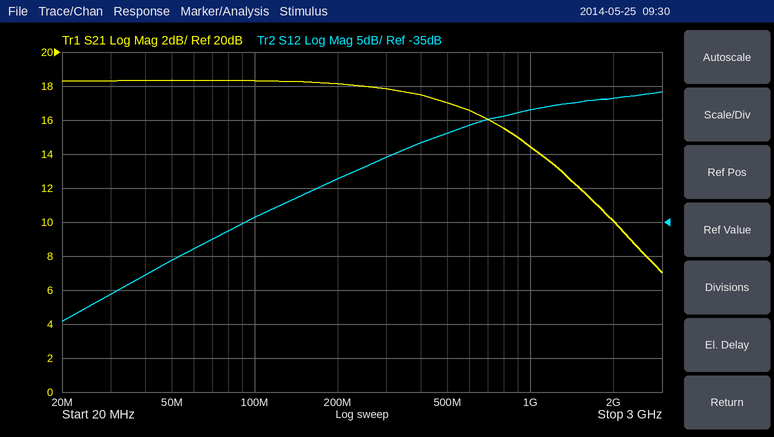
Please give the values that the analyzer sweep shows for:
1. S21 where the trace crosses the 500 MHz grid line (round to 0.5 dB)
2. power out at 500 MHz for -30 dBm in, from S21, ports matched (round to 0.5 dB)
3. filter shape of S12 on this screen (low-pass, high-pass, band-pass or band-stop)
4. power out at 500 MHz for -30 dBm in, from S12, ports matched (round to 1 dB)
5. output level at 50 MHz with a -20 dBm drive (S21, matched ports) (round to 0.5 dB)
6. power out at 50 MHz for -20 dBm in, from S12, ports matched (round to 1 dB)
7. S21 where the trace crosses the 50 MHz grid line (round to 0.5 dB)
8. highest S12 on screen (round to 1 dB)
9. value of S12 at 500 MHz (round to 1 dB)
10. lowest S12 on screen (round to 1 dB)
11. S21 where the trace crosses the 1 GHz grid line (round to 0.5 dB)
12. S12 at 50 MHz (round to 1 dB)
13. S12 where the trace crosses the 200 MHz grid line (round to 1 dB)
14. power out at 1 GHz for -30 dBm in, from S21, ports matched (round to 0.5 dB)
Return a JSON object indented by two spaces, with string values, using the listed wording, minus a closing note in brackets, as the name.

{
  "S21 where the trace crosses the 500 MHz grid line": "17.0 dB",
  "power out at 500 MHz for -30 dBm in, from S21, ports matched": "-13.0 dBm",
  "filter shape of S12 on this screen": "high-pass",
  "power out at 500 MHz for -30 dBm in, from S12, ports matched": "-52 dBm",
  "output level at 50 MHz with a -20 dBm drive (S21, matched ports)": "-1.5 dBm",
  "power out at 50 MHz for -20 dBm in, from S12, ports matched": "-61 dBm",
  "S21 where the trace crosses the 50 MHz grid line": "18.5 dB",
  "highest S12 on screen": "-16 dB",
  "value of S12 at 500 MHz": "-22 dB",
  "lowest S12 on screen": "-50 dB",
  "S21 where the trace crosses the 1 GHz grid line": "14.5 dB",
  "S12 at 50 MHz": "-41 dB",
  "S12 where the trace crosses the 200 MHz grid line": "-29 dB",
  "power out at 1 GHz for -30 dBm in, from S21, ports matched": "-15.5 dBm"
}
